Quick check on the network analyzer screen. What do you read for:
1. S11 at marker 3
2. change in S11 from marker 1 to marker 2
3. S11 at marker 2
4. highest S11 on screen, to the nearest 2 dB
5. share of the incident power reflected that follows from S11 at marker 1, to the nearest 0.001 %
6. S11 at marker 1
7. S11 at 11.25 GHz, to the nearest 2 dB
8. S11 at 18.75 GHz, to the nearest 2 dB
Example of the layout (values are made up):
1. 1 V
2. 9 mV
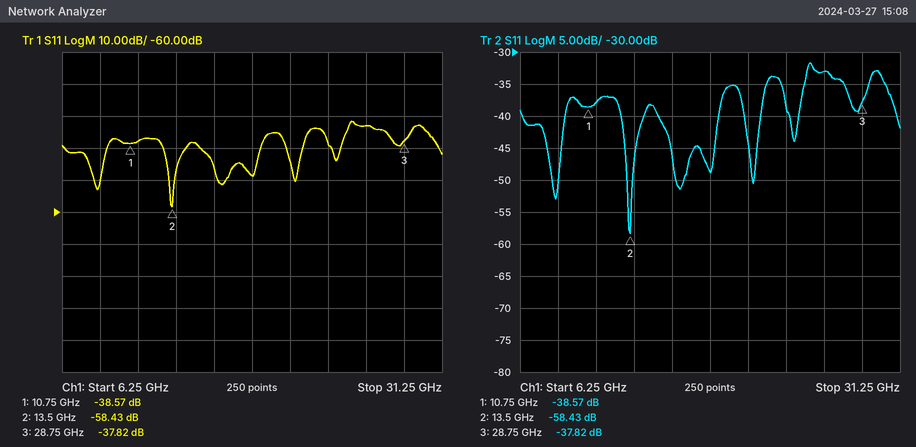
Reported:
1. -37.82 dB
2. -19.86 dB
3. -58.43 dB
4. -32 dB
5. 0.014 %
6. -38.57 dB
7. -38 dB
8. -48 dB
